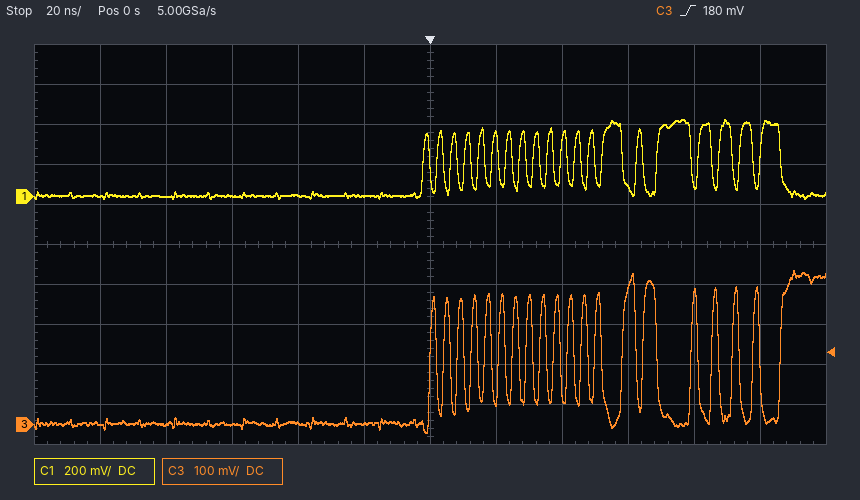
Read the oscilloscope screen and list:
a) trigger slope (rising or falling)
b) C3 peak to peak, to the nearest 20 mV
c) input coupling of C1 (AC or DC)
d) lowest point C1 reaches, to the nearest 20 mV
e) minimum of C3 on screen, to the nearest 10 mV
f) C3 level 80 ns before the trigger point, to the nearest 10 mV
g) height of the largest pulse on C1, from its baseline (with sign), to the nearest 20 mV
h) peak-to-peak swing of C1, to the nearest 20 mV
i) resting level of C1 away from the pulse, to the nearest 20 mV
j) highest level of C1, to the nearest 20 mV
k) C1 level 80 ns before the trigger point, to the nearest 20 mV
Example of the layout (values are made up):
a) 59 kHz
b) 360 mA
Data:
a) rising
b) 400 mV
c) DC
d) -20 mV
e) -20 mV
f) 0 mV
g) +380 mV
h) 400 mV
i) 0 mV
j) 380 mV
k) 0 mV
